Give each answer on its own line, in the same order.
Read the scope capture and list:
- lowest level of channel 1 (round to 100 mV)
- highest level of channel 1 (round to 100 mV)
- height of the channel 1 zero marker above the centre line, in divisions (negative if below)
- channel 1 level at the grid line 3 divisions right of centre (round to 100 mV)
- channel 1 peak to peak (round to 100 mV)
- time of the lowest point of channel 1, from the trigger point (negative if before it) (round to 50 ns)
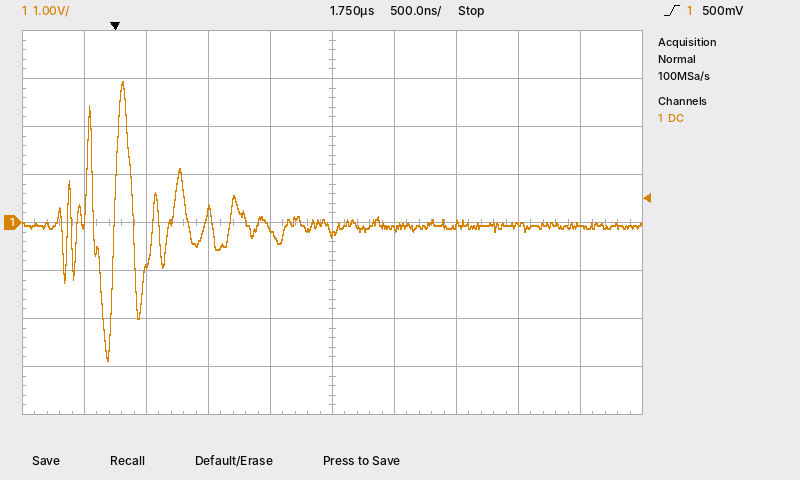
-2.9 V
2.9 V
0.0 div
0.0 V
5.8 V
-50 ns
